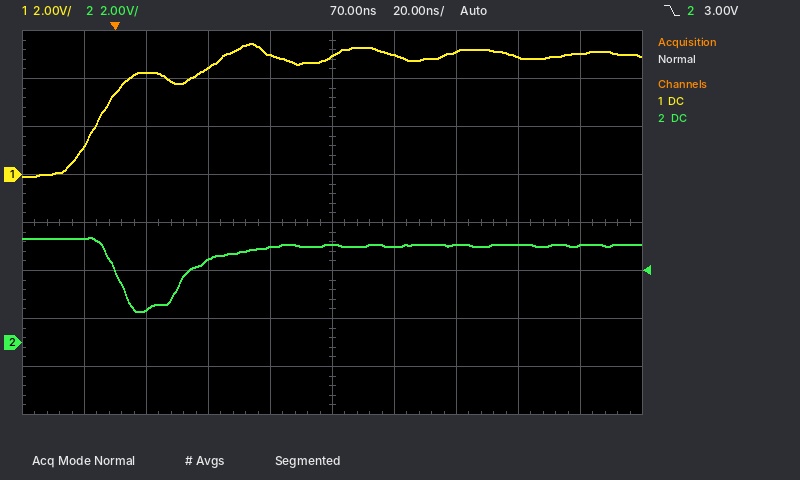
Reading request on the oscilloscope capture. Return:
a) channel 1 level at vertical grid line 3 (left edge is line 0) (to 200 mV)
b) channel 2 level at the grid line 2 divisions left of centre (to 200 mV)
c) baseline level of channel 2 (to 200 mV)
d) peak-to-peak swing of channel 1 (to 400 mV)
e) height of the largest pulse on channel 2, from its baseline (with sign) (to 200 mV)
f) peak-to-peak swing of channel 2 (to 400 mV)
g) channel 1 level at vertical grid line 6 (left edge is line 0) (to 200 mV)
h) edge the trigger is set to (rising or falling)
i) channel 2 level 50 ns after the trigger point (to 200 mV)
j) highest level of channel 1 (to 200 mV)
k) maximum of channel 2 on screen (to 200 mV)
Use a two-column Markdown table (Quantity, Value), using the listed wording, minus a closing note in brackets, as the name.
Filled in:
| Quantity | Value |
|---|---|
| channel 1 level at vertical grid line 3 (left edge is line 0) | 4.4 V |
| channel 2 level at the grid line 2 divisions left of centre | 3.4 V |
| baseline level of channel 2 | 4.0 V |
| peak-to-peak swing of channel 1 | 5.6 V |
| height of the largest pulse on channel 2, from its baseline (with sign) | -2.8 V |
| peak-to-peak swing of channel 2 | 3.2 V |
| channel 1 level at vertical grid line 6 (left edge is line 0) | 5.0 V |
| edge the trigger is set to | falling |
| channel 2 level 50 ns after the trigger point | 4.0 V |
| highest level of channel 1 | 5.4 V |
| maximum of channel 2 on screen | 4.4 V |
